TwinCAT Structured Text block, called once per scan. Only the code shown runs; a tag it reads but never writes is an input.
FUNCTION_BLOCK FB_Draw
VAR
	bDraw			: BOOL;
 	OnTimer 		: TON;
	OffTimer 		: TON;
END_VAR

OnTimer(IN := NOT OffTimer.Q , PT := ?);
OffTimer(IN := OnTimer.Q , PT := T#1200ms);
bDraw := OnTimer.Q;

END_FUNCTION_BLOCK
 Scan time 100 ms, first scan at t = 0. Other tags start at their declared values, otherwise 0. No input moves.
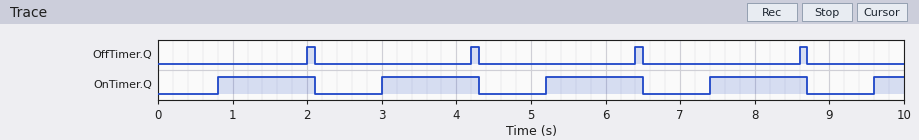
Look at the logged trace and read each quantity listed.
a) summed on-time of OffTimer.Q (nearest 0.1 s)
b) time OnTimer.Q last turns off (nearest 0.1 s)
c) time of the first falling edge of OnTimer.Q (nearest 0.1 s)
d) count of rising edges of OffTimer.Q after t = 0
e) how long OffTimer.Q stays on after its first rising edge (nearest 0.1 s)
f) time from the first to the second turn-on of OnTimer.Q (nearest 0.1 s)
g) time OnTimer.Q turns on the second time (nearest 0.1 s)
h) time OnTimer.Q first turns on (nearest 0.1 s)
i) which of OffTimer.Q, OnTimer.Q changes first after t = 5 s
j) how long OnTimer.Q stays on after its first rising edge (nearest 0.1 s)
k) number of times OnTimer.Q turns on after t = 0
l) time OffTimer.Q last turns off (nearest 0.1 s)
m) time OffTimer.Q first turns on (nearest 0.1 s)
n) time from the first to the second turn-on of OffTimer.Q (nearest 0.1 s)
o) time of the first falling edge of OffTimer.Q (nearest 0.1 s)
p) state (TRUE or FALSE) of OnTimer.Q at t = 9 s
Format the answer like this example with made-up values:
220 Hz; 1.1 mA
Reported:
0.4 s; 8.7 s; 2.1 s; 4; 0.1 s; 2.2 s; 3.0 s; 0.8 s; OnTimer.Q; 1.3 s; 5; 8.7 s; 2.0 s; 2.2 s; 2.1 s; FALSE
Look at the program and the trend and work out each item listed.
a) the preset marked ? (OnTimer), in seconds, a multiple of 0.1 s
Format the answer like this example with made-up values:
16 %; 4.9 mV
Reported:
0.8 s
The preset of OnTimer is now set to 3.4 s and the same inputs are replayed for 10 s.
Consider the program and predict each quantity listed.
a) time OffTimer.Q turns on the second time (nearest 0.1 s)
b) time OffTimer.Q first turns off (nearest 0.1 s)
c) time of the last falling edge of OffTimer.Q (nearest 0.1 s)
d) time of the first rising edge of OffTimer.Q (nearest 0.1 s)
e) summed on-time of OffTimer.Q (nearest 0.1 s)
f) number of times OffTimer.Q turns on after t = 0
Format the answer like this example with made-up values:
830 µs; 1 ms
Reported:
9.4 s; 4.7 s; 9.5 s; 4.6 s; 0.2 s; 2
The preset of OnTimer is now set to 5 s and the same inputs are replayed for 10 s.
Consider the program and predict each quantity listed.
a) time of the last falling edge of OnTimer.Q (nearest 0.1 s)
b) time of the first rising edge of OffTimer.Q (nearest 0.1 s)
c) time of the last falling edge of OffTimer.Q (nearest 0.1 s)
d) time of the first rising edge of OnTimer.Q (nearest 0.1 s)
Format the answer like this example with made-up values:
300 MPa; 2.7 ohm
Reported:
6.3 s; 6.2 s; 6.3 s; 5.0 s
